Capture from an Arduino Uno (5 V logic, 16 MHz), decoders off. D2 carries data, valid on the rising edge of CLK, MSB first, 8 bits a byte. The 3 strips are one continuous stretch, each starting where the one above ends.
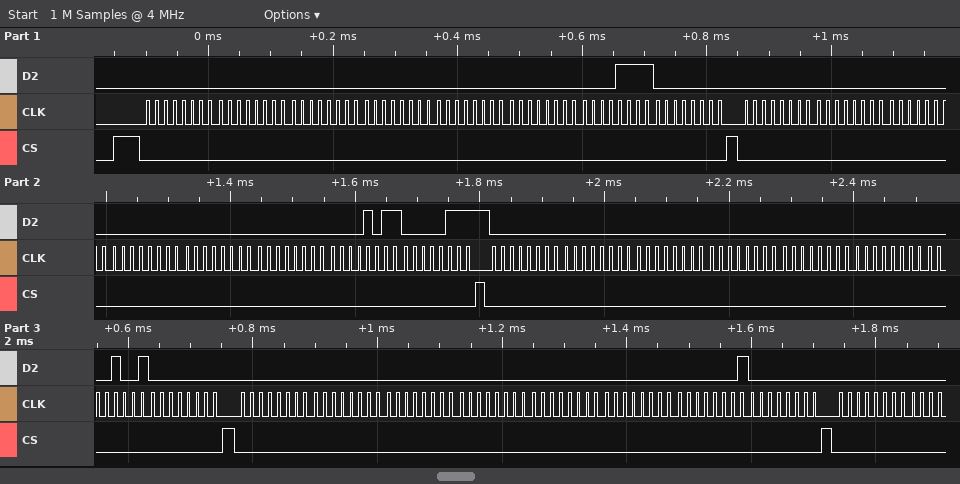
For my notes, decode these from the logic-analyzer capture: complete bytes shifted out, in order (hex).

0x00 0x00 0x00 0x00 0x00 0x00 0x0F 0x00 0x00 0x00 0x00 0x00 0x00 0x00 0x0B 0x07 0x00 0x00 0x00 0x00 0x00 0x00 0x09 0x00 0x00 0x00 0x00 0x00 0x00 0x00 0x01 0x00 0x00
